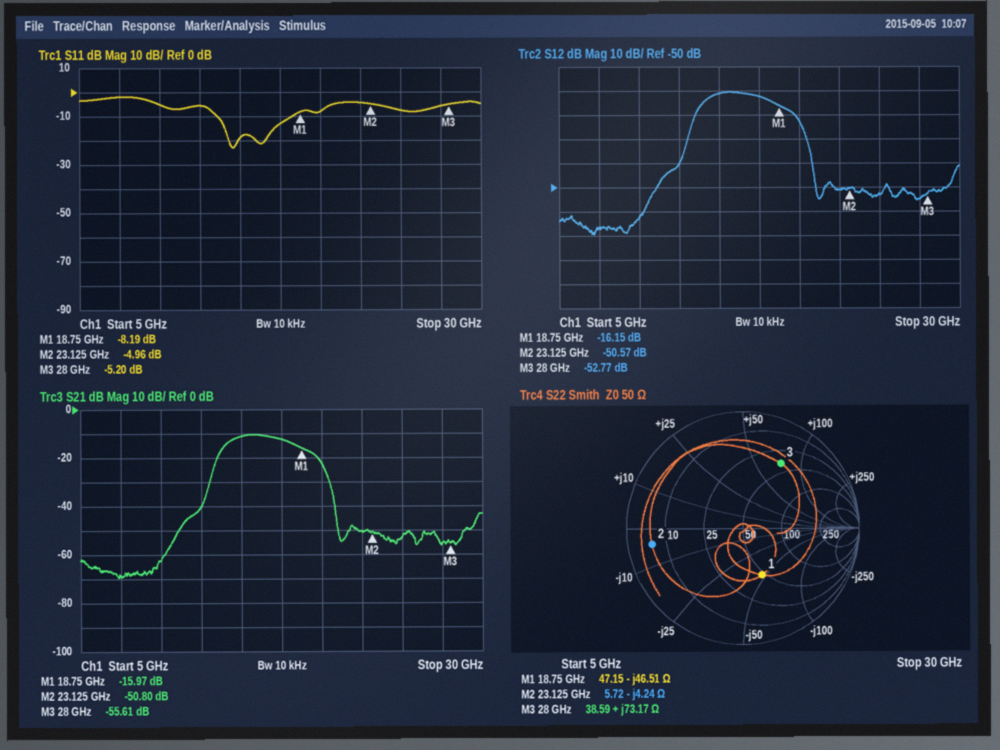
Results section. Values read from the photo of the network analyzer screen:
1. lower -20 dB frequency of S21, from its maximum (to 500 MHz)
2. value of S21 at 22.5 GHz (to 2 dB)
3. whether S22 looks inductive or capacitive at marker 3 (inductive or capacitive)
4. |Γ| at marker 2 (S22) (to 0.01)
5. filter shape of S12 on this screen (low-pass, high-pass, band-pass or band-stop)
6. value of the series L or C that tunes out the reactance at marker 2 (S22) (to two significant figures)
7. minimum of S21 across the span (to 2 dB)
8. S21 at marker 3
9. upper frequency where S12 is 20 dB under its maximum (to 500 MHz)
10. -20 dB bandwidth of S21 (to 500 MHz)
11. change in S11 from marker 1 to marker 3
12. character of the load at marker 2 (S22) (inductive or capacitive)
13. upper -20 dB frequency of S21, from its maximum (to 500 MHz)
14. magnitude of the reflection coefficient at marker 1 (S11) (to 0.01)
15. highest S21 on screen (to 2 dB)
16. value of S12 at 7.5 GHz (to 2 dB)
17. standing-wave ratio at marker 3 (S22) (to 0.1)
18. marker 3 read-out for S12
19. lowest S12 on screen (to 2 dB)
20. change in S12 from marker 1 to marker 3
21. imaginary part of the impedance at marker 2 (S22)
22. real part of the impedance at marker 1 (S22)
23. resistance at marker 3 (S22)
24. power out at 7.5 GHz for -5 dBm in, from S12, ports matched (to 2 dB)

13.0 GHz
-50 dB
inductive
0.80
band-pass
29 pH
-70 dB
-55.61 dB
20.5 GHz
7.5 GHz
2.99 dB
capacitive
20.5 GHz
0.39
-10 dB
-66 dB
4.6
-52.77 dB
-70 dB
-36.62 dB
-4.24 Ω
47.15 Ω
38.59 Ω
-72 dBm
